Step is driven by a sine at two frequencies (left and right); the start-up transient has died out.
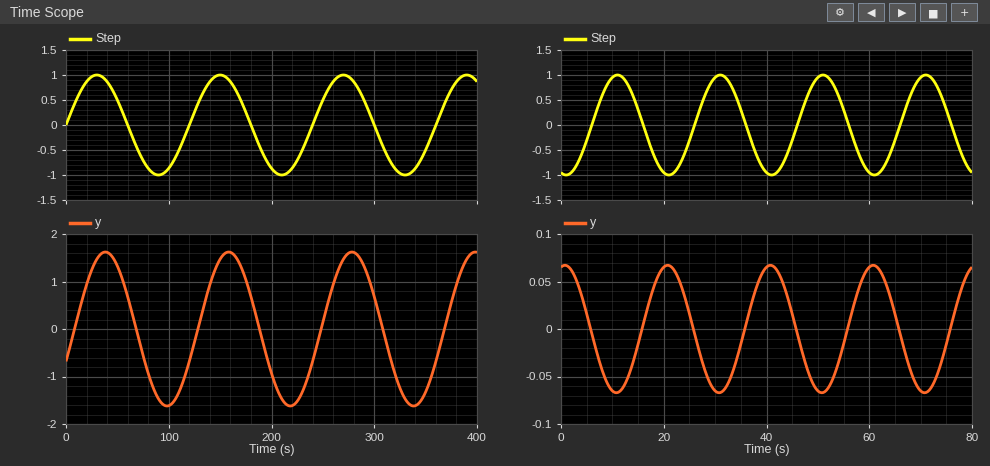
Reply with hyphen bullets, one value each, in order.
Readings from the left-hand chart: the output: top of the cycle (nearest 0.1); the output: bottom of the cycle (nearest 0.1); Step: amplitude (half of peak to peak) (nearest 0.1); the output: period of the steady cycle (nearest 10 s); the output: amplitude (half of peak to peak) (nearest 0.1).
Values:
- 1.6
- -1.6
- 1.0
- 120 s
- 1.6
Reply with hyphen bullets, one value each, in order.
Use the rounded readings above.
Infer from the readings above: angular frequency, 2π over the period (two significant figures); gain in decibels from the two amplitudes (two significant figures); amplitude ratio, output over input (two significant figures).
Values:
- 0.052 rad/s
- 4.1 dB
- 1.6
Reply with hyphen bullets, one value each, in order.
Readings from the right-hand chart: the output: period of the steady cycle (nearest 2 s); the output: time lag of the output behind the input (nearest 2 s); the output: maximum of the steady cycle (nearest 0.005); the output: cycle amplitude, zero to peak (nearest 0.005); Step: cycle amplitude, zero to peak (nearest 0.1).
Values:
- 20 s
- 10 s
- 0.065
- 0.065
- 1.0
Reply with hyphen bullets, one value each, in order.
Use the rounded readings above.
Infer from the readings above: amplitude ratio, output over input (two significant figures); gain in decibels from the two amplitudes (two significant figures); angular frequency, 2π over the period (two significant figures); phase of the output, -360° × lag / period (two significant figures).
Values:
- 0.065
- -24 dB
- 0.31 rad/s
- -180°
